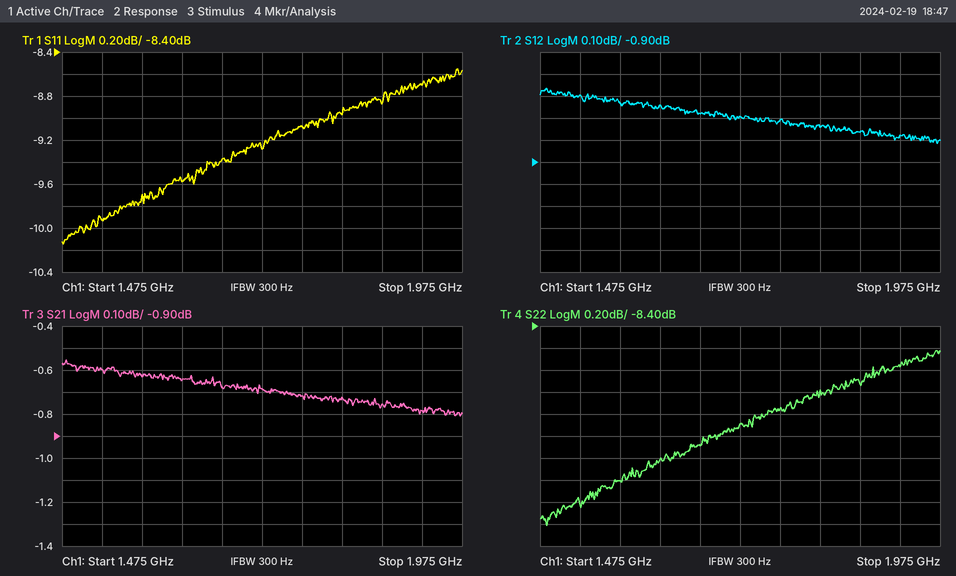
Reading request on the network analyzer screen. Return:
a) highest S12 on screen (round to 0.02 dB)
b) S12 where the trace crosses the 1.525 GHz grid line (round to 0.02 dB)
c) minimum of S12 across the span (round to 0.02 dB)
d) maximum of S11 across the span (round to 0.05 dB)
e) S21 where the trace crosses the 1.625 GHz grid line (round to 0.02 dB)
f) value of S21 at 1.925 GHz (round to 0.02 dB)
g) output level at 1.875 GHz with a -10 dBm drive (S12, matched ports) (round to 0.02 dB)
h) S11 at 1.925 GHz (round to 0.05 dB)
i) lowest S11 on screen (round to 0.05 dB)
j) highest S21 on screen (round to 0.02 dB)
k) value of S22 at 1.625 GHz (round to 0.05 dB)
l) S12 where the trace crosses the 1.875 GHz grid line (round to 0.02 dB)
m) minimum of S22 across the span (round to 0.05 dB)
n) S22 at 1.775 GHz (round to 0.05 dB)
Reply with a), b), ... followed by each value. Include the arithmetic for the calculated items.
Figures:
a) -0.56 dB
b) -0.60 dB
c) -0.82 dB
d) -8.55 dB
e) -0.64 dB
f) -0.78 dB
g) -10 dBm + (-0.76 dB) = -10.76 dBm
h) -8.70 dB
i) -10.15 dB
j) -0.56 dB
k) -9.60 dB
l) -0.76 dB
m) -10.20 dB
n) -9.15 dB
